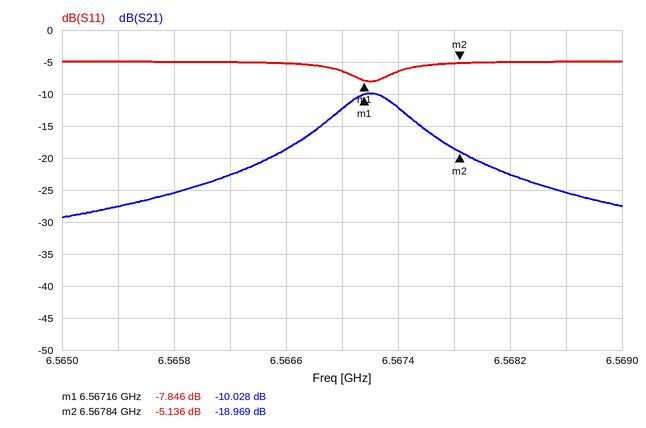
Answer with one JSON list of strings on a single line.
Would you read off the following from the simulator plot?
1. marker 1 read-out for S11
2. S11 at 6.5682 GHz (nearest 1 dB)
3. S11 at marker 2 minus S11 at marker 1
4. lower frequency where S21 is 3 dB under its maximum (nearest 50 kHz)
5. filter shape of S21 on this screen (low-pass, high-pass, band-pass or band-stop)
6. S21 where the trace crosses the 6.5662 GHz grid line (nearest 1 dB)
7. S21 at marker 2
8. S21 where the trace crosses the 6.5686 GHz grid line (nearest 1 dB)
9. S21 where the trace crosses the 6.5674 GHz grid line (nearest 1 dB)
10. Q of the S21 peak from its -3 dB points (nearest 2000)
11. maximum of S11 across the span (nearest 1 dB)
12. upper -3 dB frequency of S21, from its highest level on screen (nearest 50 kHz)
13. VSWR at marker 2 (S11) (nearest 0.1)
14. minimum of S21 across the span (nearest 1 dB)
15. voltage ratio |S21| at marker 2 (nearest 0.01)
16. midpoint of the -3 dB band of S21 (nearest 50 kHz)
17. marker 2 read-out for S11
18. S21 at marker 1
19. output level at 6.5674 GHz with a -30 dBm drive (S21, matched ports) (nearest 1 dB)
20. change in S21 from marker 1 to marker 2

["-7.846 dB", "-5 dB", "2.710 dB", "6.56695 GHz", "band-pass", "-23 dB", "-18.969 dB", "-25 dB", "-12 dB", "14000", "-5 dB", "6.56745 GHz", "3.5", "-29 dB", "0.11", "6.56720 GHz", "-5.136 dB", "-10.028 dB", "-42 dBm", "-8.941 dB"]
